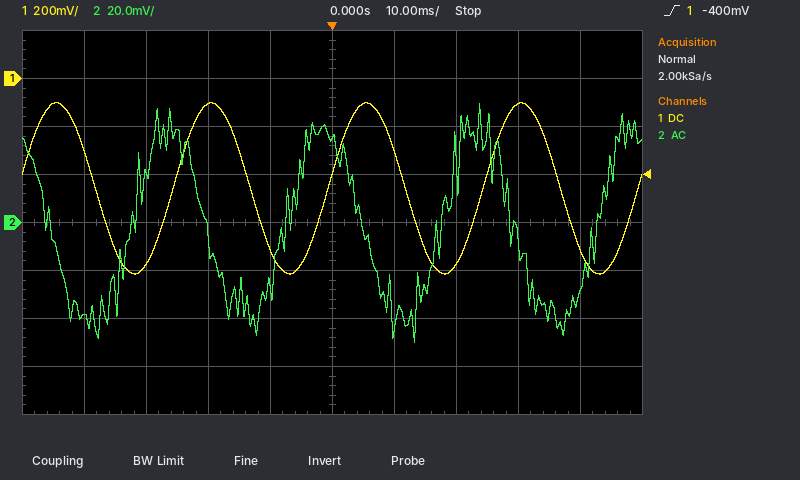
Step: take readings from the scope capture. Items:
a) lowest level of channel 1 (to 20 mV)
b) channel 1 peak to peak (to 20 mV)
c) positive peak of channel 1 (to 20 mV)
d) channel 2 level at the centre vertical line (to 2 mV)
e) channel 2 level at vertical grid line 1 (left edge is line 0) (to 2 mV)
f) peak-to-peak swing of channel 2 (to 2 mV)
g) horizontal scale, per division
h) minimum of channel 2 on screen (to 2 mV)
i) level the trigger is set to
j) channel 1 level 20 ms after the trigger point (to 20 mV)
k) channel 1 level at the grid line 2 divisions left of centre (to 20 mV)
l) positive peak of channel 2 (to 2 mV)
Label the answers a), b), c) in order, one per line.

a) -820 mV
b) 720 mV
c) -100 mV
d) 36 mV
e) -40 mV
f) 100 mV
g) 10 ms
h) -50 mV
i) -400 mV
j) -780 mV
k) -100 mV
l) 50 mV
